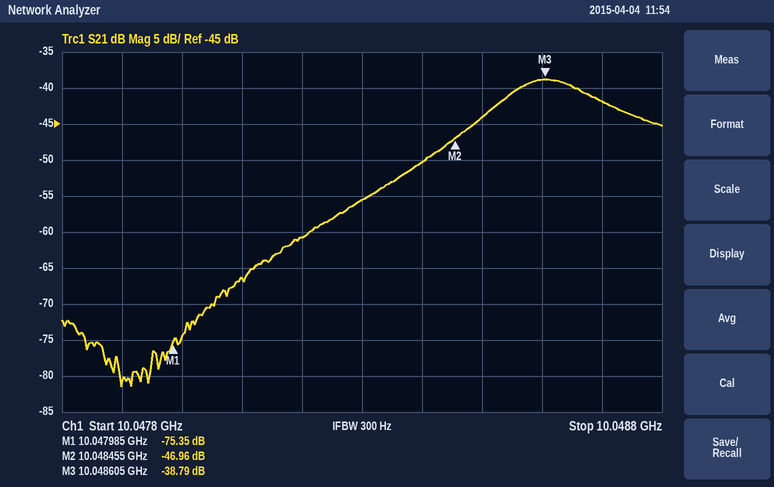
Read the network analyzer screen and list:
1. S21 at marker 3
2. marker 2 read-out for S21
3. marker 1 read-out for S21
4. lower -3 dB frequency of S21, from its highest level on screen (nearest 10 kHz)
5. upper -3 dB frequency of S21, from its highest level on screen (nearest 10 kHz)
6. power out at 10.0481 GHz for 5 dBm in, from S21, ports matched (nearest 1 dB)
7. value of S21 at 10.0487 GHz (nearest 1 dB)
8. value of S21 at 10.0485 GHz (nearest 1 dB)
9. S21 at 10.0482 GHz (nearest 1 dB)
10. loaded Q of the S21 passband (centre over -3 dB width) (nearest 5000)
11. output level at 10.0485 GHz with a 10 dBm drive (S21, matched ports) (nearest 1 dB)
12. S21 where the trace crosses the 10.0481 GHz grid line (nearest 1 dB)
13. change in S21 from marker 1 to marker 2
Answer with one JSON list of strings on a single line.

["-38.79 dB", "-46.96 dB", "-75.35 dB", "10.04853 GHz", "10.04870 GHz", "-61 dBm", "-42 dB", "-44 dB", "-61 dB", "60000", "-34 dBm", "-66 dB", "28.39 dB"]
